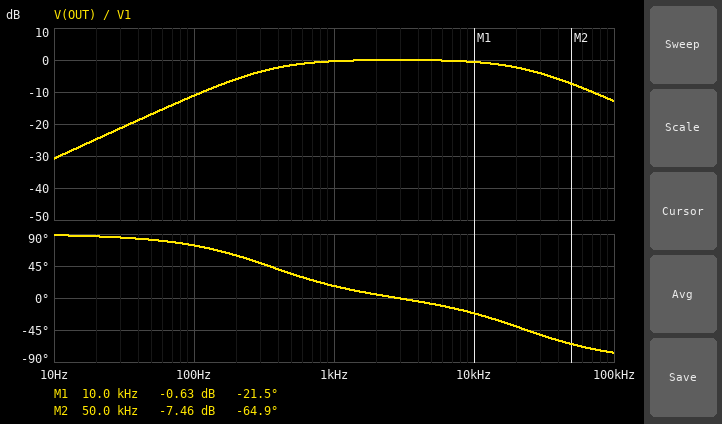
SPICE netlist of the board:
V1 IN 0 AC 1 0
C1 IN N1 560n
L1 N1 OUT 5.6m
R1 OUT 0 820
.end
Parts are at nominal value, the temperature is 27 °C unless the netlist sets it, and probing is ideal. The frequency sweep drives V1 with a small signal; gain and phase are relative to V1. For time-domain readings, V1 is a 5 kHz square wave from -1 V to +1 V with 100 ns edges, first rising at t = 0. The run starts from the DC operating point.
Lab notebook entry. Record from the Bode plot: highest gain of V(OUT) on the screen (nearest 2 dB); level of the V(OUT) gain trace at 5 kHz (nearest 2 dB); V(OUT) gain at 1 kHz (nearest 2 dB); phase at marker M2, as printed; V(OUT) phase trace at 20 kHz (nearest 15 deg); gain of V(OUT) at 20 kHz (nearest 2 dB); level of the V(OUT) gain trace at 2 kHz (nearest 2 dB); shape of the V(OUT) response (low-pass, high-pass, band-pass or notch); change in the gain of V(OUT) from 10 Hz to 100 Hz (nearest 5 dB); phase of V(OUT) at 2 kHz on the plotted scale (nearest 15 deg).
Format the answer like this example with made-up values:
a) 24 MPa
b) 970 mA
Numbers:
a) 0 dB
b) 0 dB
c) 0 dB
d) -64.9 deg
e) -45 deg
f) -2 dB
g) 0 dB
h) band-pass
i) 20 dB
j) 0 deg
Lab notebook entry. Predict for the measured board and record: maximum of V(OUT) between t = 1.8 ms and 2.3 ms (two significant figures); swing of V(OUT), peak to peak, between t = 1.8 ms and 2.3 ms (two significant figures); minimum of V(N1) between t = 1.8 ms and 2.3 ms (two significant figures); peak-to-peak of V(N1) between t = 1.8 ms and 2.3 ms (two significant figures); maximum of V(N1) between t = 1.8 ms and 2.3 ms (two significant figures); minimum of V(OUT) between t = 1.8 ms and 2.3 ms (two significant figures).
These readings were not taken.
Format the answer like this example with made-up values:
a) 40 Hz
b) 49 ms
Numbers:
a) 1.1 V
b) 2.1 V
c) -1.1 V
d) 2.2 V
e) 1.1 V
f) -1.0 V
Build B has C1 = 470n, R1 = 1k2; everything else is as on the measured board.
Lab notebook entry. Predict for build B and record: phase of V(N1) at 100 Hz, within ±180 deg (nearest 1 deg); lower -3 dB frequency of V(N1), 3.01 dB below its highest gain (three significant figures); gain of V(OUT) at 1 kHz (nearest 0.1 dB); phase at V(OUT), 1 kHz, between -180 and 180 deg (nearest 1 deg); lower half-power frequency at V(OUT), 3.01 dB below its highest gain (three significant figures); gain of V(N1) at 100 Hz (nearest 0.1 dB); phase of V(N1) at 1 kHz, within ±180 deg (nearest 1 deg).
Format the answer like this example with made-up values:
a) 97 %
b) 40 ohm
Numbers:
a) 71 deg
b) 284 Hz
c) -0.3 dB
d) 14 deg
e) 280 Hz
f) -9.5 dB
g) 16 deg
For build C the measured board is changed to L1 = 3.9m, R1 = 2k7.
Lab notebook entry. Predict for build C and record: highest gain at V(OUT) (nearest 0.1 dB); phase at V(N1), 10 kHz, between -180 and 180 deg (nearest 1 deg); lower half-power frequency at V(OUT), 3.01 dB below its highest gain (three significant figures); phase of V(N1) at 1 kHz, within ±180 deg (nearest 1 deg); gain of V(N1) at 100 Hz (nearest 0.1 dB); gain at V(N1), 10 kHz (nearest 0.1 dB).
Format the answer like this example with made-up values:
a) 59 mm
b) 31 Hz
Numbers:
a) 0 dB
b) 1 deg
c) 105 Hz
d) 6 deg
e) -3.2 dB
f) 0 dB
